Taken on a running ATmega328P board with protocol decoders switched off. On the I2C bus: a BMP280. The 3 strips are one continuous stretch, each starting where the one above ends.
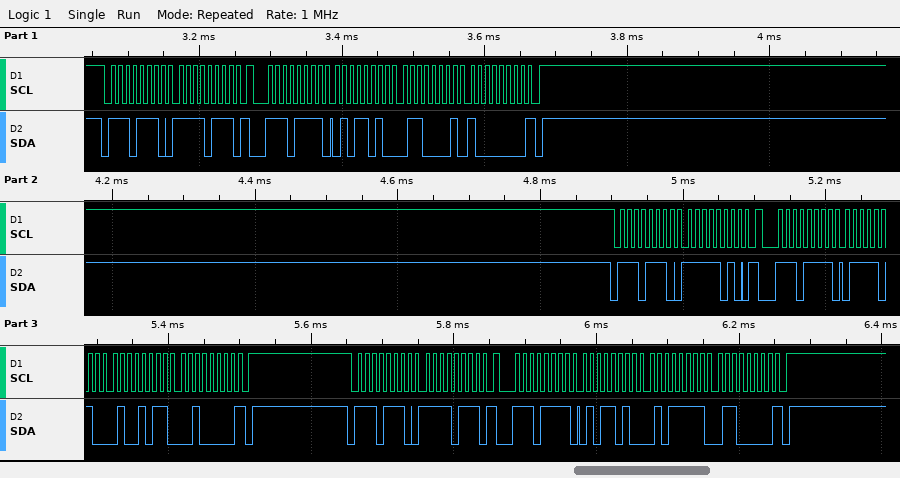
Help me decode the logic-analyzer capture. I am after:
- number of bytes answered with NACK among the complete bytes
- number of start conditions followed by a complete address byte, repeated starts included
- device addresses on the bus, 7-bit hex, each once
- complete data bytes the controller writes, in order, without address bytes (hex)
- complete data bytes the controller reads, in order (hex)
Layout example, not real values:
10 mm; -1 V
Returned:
3; 6; 0x77; F7 FA F7; 5A 61 80 7A 4B 20 5A 5F 60
